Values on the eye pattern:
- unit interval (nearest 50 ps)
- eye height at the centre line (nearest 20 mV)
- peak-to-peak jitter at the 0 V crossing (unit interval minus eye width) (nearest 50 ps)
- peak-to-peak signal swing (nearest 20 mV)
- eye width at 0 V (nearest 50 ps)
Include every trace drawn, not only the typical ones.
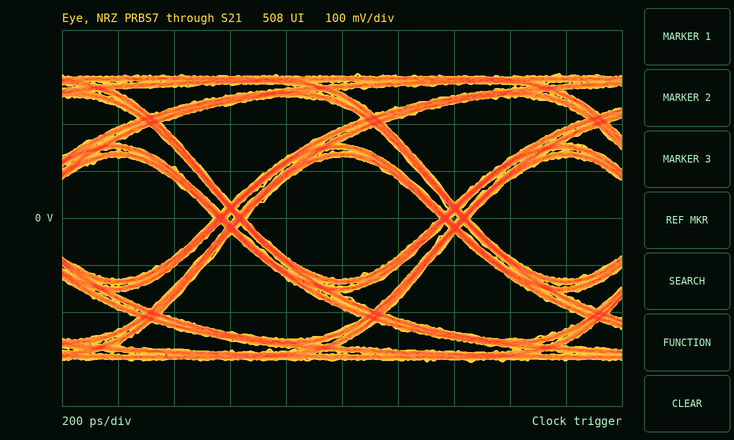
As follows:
800 ps
260 mV
100 ps
620 mV
700 ps
